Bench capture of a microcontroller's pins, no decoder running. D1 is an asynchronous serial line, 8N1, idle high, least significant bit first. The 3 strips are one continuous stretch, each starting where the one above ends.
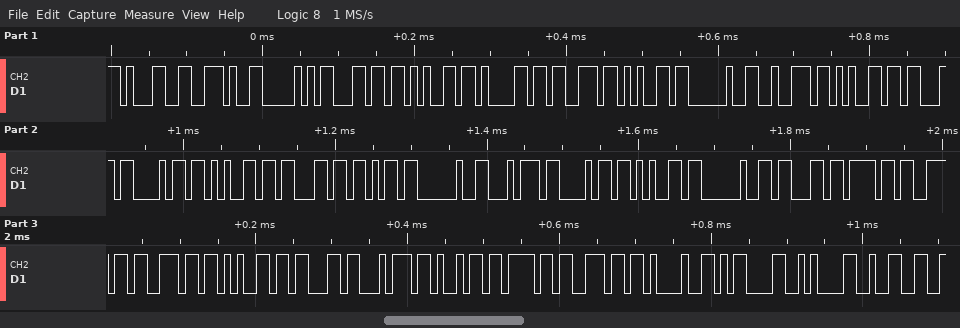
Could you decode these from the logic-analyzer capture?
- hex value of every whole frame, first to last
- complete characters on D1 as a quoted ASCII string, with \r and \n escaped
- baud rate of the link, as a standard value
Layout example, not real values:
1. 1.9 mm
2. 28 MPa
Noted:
1. 31 2E 50 6C 65 61 73 65 20 72 65 63 68 65 63 6B 20 74 68 65 20 63 6F 6E 6E 65 63 74 69 6F 6E 21 0D 0A 32
2. "1.Please recheck the connection!\r\n2"
3. 115200 baud
